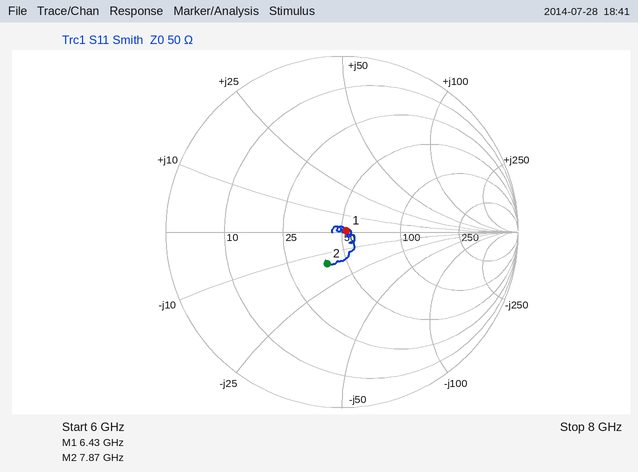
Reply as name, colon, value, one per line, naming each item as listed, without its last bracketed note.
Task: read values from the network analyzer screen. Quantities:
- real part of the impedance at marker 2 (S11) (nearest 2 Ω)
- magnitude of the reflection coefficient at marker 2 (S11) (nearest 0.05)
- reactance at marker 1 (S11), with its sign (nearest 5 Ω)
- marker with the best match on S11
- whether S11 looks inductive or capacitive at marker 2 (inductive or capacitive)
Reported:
real part of the impedance at marker 2 (S11): 40 Ω
magnitude of the reflection coefficient at marker 2 (S11): 0.20
reactance at marker 1 (S11), with its sign: 0 Ω
marker with the best match on S11: marker 1
whether S11 looks inductive or capacitive at marker 2: capacitive
